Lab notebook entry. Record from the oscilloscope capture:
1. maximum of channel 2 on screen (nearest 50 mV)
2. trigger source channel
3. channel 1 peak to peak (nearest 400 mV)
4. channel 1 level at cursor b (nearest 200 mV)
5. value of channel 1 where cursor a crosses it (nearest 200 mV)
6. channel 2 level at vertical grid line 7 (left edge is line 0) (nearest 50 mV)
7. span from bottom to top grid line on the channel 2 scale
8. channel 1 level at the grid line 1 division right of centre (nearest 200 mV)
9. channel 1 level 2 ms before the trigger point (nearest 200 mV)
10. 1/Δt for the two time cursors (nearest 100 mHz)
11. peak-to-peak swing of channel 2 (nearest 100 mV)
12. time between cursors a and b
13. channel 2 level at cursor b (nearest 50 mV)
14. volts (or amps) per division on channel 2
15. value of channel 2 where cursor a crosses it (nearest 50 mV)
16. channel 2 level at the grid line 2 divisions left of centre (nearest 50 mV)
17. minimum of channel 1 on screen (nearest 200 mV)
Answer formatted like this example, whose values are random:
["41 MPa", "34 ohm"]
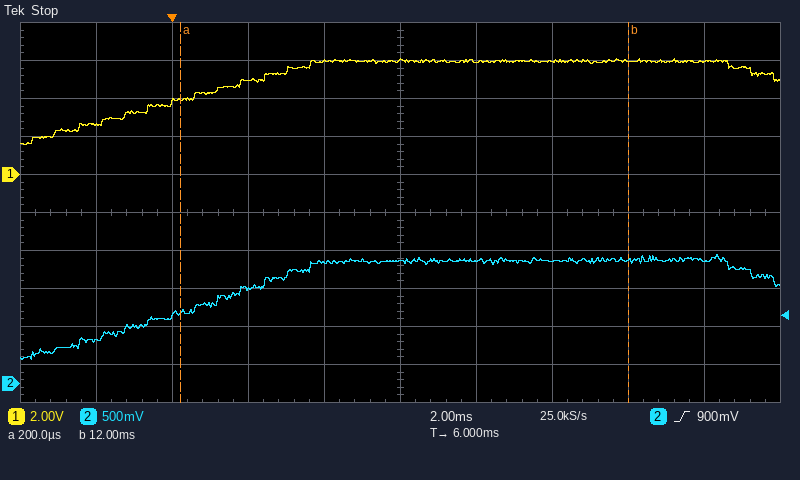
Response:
["1.70 V", "channel 2", "4.4 V", "6.0 V", "4.0 V", "1.60 V", "5 V", "6.0 V", "2.6 V", "84.7 Hz", "1.40 V", "11.8 ms", "1.60 V", "500 mV", "950 mV", "1.25 V", "1.6 V"]
